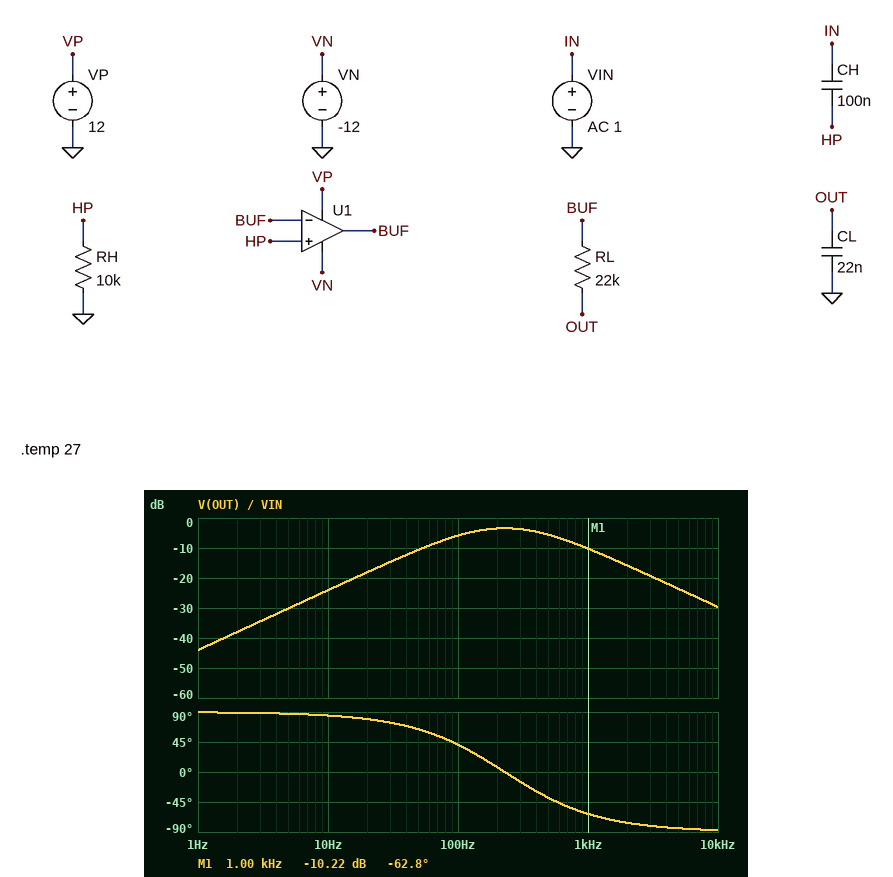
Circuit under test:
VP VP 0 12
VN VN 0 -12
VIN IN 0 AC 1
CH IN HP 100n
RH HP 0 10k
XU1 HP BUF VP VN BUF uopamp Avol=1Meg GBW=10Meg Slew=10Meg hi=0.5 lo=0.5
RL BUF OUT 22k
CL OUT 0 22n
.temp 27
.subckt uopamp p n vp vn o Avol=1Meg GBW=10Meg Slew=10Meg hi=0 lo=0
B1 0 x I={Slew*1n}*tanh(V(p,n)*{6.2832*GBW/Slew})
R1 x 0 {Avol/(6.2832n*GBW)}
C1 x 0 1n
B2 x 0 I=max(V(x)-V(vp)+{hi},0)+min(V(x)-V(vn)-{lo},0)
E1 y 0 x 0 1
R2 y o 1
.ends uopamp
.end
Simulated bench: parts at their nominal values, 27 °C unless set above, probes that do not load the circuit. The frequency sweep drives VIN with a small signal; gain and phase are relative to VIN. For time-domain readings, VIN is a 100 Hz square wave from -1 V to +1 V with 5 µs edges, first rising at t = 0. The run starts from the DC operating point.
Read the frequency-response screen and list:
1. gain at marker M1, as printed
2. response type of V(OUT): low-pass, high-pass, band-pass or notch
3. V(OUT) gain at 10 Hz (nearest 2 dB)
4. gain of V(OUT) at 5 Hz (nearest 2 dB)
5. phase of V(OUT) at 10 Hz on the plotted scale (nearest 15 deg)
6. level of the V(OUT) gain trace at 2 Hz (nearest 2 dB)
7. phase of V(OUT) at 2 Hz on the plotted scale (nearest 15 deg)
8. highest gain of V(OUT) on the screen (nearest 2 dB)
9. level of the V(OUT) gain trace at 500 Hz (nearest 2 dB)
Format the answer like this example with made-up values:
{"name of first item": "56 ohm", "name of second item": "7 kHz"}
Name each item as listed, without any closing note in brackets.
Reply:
{"gain at marker M1, as printed": "-10.22 dB", "response type of V(OUT): low-pass, high-pass, band-pass or notch": "band-pass", "V(OUT) gain at 10 Hz": "-24 dB", "gain of V(OUT) at 5 Hz": "-30 dB", "phase of V(OUT) at 10 Hz on the plotted scale": "90 deg", "level of the V(OUT) gain trace at 2 Hz": "-38 dB", "phase of V(OUT) at 2 Hz on the plotted scale": "90 deg", "highest gain of V(OUT) on the screen": "-4 dB", "level of the V(OUT) gain trace at 500 Hz": "-6 dB"}
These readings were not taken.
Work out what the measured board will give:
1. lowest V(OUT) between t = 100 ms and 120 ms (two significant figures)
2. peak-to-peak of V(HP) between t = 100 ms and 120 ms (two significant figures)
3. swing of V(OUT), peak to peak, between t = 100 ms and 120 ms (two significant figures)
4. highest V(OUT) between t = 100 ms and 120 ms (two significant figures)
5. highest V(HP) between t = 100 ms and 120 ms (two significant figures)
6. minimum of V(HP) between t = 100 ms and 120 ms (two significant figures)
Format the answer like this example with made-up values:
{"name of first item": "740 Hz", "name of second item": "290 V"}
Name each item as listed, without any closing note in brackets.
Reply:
{"lowest V(OUT) between t = 100 ms and 120 ms": "-1.0 V", "peak-to-peak of V(HP) between t = 100 ms and 120 ms": "4.0 V", "swing of V(OUT), peak to peak, between t = 100 ms and 120 ms": "2.0 V", "highest V(OUT) between t = 100 ms and 120 ms": "1.0 V", "highest V(HP) between t = 100 ms and 120 ms": "2.0 V", "minimum of V(HP) between t = 100 ms and 120 ms": "-2.0 V"}
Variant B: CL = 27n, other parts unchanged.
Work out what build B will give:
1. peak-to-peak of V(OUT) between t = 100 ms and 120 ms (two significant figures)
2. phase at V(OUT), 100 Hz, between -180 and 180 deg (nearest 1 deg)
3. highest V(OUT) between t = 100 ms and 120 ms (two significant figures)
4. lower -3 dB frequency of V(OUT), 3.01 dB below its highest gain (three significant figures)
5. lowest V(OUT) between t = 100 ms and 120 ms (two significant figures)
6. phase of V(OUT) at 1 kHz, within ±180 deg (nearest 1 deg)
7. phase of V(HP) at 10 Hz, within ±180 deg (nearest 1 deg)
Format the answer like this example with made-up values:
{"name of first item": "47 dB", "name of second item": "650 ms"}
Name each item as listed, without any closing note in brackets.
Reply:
{"peak-to-peak of V(OUT) between t = 100 ms and 120 ms": "1.8 V", "phase at V(OUT), 100 Hz, between -180 and 180 deg": "37 deg", "highest V(OUT) between t = 100 ms and 120 ms": "920 mV", "lower -3 dB frequency of V(OUT), 3.01 dB below its highest gain": "83.5 Hz", "lowest V(OUT) between t = 100 ms and 120 ms": "-920 mV", "phase of V(OUT) at 1 kHz, within ±180 deg": "-66 deg", "phase of V(HP) at 10 Hz, within ±180 deg": "86 deg"}
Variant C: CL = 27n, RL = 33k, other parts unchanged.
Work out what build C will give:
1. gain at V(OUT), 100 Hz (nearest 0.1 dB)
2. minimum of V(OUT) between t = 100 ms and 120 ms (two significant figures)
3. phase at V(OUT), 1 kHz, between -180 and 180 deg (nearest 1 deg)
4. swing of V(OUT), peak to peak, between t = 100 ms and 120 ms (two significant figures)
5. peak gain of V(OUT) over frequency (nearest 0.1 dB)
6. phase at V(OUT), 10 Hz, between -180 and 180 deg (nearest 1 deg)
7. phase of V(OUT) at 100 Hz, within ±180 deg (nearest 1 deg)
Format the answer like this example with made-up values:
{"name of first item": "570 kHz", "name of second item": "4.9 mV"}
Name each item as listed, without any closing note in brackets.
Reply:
{"gain at V(OUT), 100 Hz": "-6.7 dB", "minimum of V(OUT) between t = 100 ms and 120 ms": "-750 mV", "phase at V(OUT), 1 kHz, between -180 and 180 deg": "-71 deg", "swing of V(OUT), peak to peak, between t = 100 ms and 120 ms": "1.5 V", "peak gain of V(OUT) over frequency": "-5.5 dB", "phase at V(OUT), 10 Hz, between -180 and 180 deg": "83 deg", "phase of V(OUT) at 100 Hz, within ±180 deg": "29 deg"}
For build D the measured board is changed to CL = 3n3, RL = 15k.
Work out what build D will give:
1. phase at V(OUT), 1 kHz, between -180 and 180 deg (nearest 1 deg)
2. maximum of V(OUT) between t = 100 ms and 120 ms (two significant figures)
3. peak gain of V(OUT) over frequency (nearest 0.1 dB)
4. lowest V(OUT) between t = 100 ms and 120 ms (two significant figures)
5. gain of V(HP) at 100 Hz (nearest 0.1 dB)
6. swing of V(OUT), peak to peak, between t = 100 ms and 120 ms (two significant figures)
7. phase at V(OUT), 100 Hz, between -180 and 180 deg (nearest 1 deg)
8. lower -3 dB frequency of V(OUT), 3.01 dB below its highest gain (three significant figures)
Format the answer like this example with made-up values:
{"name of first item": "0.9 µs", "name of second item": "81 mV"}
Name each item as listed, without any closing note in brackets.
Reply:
{"phase at V(OUT), 1 kHz, between -180 and 180 deg": "-8 deg", "maximum of V(OUT) between t = 100 ms and 120 ms": "1.7 V", "peak gain of V(OUT) over frequency": "-0.4 dB", "lowest V(OUT) between t = 100 ms and 120 ms": "-1.7 V", "gain of V(HP) at 100 Hz": "-5.5 dB", "swing of V(OUT), peak to peak, between t = 100 ms and 120 ms": "3.4 V", "phase at V(OUT), 100 Hz, between -180 and 180 deg": "56 deg", "lower -3 dB frequency of V(OUT), 3.01 dB below its highest gain": "145 Hz"}
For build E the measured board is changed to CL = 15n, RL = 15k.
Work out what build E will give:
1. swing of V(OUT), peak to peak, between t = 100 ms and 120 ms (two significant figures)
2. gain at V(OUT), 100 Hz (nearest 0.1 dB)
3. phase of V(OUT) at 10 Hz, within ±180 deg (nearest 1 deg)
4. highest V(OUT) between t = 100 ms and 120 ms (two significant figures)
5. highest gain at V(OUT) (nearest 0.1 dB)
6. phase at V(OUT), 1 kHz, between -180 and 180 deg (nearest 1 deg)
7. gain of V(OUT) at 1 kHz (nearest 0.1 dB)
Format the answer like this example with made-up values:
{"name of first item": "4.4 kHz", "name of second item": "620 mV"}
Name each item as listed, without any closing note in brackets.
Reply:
{"swing of V(OUT), peak to peak, between t = 100 ms and 120 ms": "2.6 V", "gain at V(OUT), 100 Hz": "-5.6 dB", "phase of V(OUT) at 10 Hz, within ±180 deg": "86 deg", "highest V(OUT) between t = 100 ms and 120 ms": "1.3 V", "highest gain at V(OUT)": "-1.8 dB", "phase at V(OUT), 1 kHz, between -180 and 180 deg": "-46 deg", "gain of V(OUT) at 1 kHz": "-4.9 dB"}
